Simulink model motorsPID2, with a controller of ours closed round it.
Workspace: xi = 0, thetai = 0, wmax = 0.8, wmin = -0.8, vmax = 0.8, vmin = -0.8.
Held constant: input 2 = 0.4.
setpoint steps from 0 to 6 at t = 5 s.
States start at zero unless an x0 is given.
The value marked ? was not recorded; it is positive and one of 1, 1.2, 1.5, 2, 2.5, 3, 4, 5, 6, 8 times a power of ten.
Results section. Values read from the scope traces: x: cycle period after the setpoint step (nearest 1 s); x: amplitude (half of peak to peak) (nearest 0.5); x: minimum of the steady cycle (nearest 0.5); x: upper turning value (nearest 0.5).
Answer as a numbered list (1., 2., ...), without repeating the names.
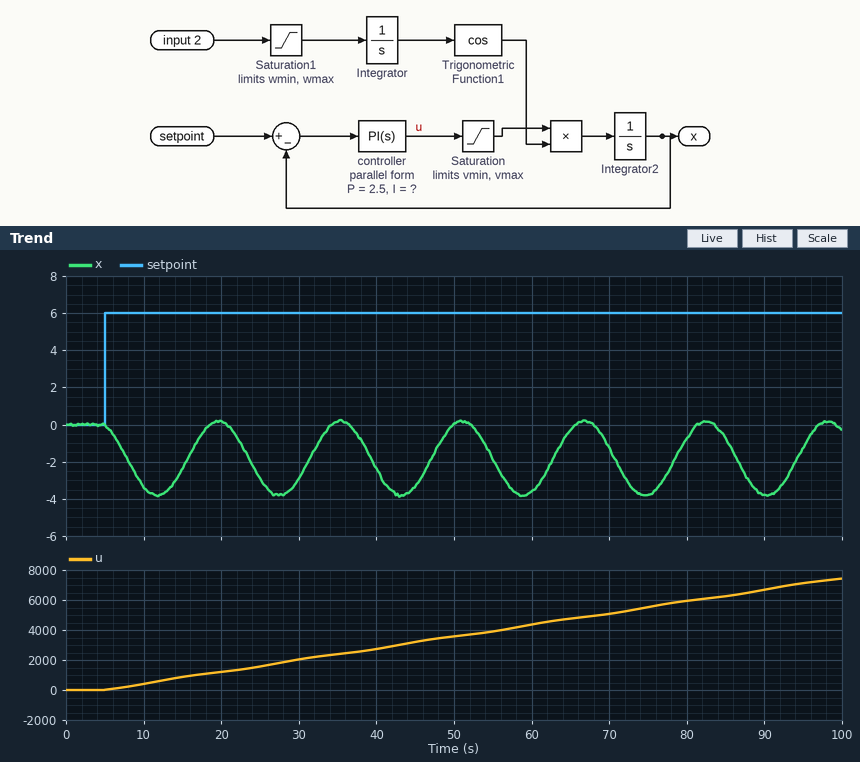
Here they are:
1. 16 s
2. 2.0
3. -4.0
4. 0.0
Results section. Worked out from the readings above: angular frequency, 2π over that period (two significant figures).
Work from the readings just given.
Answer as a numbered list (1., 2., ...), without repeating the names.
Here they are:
1. 0.39 rad/s
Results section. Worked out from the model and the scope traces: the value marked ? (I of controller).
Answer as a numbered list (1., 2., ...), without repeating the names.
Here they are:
1. 10
